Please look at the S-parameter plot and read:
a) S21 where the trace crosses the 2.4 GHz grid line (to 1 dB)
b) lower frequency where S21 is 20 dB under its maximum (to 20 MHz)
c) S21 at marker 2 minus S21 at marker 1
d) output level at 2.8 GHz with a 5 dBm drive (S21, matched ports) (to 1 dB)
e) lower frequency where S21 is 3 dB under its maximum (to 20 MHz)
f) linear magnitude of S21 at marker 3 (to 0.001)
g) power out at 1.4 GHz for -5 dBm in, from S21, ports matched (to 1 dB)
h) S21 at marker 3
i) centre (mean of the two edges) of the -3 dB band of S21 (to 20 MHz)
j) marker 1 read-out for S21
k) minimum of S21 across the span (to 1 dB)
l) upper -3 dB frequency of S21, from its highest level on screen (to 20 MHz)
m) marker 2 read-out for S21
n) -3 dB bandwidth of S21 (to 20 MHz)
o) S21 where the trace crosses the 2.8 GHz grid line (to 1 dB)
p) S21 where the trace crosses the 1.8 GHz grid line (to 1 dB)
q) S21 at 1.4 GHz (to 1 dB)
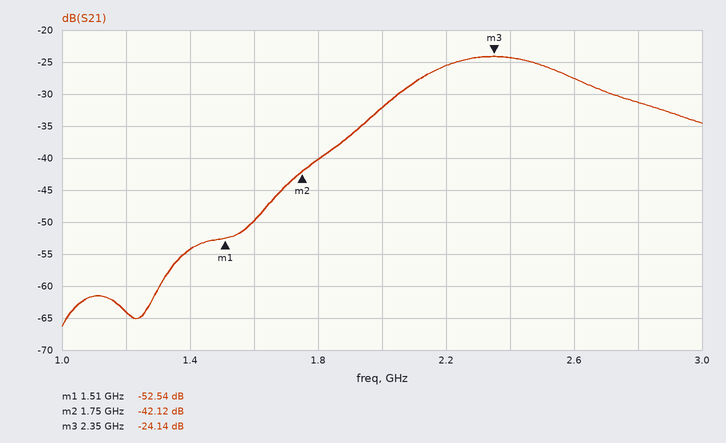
-24 dB
1.70 GHz
10.42 dB
-26 dBm
2.14 GHz
0.062
-59 dBm
-24.14 dB
2.36 GHz
-52.54 dB
-66 dB
2.58 GHz
-42.12 dB
440 MHz
-31 dB
-40 dB
-54 dB
